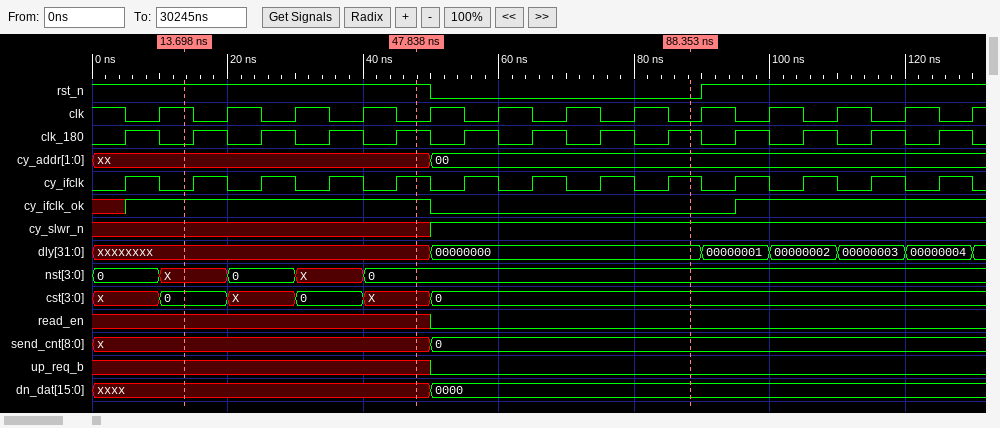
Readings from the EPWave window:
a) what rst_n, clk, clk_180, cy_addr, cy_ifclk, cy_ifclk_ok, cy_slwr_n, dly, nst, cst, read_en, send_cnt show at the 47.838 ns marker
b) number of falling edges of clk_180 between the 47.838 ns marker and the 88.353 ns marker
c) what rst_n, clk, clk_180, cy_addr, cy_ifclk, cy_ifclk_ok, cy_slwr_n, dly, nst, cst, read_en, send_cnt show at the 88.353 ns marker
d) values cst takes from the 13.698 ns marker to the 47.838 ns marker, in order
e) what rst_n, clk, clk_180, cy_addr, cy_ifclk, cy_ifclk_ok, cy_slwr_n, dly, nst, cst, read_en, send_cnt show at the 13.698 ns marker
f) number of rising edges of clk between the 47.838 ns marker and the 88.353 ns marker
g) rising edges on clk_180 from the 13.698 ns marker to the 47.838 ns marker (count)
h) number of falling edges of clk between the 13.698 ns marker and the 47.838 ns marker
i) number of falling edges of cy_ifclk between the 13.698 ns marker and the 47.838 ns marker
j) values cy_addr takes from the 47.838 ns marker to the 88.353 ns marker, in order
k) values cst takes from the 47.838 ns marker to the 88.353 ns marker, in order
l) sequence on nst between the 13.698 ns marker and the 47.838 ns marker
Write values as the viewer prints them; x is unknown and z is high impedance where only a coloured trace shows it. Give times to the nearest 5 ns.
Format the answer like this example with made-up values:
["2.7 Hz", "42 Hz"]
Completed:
["rst_n=1, clk=0, clk_180=1, cy_addr=xx, cy_ifclk=1, cy_ifclk_ok=1, cy_slwr_n=x, dly=xxxxxxxx, nst=0, cst=X, read_en=x, send_cnt=x", "4", "rst_n=0, clk=0, clk_180=1, cy_addr=00, cy_ifclk=1, cy_ifclk_ok=0, cy_slwr_n=1, dly=00000000, nst=0, cst=0, read_en=0, send_cnt=0", "0, X, 0, X", "rst_n=1, clk=1, clk_180=0, cy_addr=xx, cy_ifclk=0, cy_ifclk_ok=1, cy_slwr_n=x, dly=xxxxxxxx, nst=X, cst=0, read_en=x, send_cnt=x", "4", "4", "4", "3", "xx, 00", "X, 0", "X, 0, X, 0"]
